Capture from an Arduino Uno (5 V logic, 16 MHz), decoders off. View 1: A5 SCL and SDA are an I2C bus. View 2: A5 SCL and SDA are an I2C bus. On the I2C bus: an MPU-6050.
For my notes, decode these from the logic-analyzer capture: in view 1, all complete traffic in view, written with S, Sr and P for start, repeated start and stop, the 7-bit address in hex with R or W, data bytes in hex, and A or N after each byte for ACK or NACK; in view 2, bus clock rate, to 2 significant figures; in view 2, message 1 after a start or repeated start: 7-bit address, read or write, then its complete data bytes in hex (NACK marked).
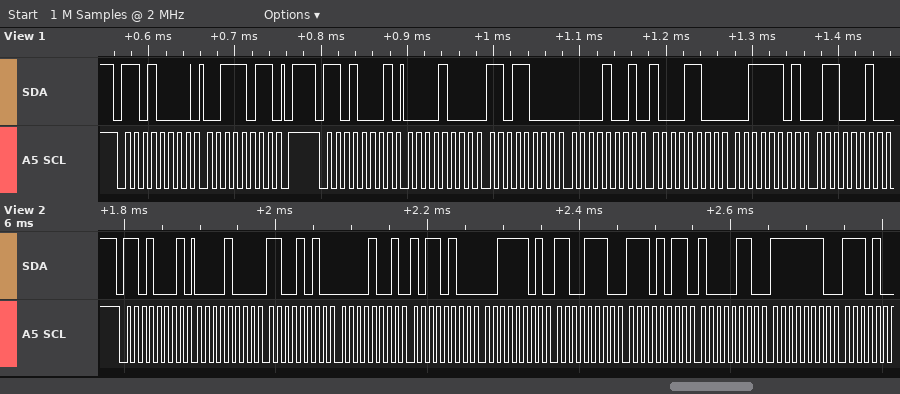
S 68W A 3B A P S 68R A 08 A D8 A 09 A 8C A 3D A 62 A
100 kHz
0x68 read: 08 CA 09 B4 3D CE EB 86 FE
